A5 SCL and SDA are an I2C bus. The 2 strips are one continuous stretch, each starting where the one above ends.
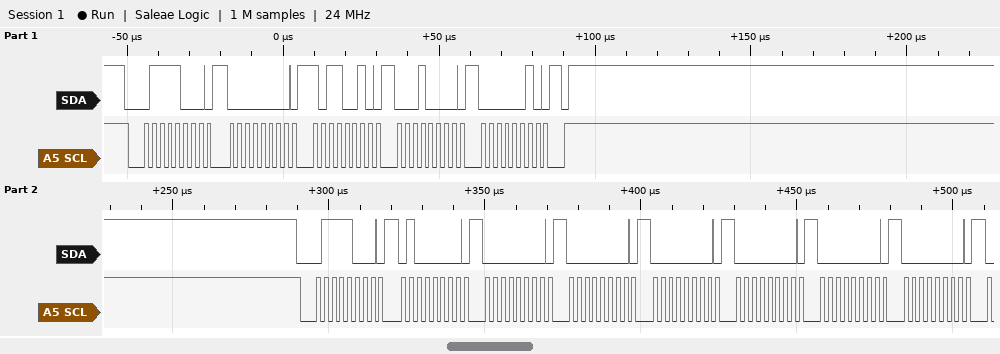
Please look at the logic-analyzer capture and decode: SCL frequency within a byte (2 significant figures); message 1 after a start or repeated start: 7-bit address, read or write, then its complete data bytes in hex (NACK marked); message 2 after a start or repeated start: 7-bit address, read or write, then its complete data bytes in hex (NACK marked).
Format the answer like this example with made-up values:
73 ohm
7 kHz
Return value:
400 kHz
0x3C write: 00 B2 10 02
0x3C write: 40 00 00 00 00 00 00
